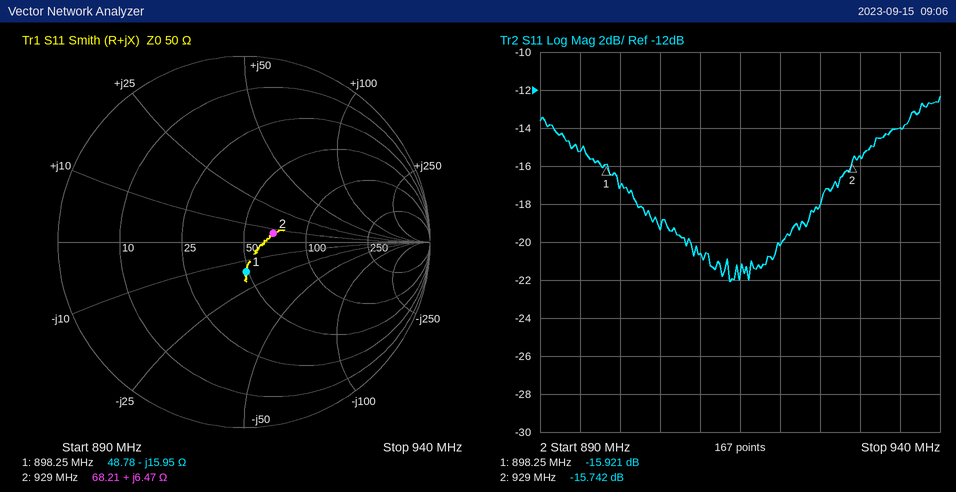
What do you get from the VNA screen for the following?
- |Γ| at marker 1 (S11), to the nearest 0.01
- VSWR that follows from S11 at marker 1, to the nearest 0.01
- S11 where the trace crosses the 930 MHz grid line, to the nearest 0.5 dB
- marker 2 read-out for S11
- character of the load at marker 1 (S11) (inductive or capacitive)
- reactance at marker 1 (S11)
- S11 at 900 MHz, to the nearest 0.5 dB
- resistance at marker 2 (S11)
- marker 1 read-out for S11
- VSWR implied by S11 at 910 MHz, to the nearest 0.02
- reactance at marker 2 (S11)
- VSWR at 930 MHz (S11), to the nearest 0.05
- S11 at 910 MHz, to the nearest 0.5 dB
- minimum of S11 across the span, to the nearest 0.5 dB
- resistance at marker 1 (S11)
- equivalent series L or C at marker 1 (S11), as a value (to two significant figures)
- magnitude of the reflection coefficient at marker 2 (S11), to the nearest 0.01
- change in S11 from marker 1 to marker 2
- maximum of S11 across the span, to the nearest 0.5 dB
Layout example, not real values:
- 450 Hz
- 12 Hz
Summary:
- 0.16
- 1.38
- -15.5 dB
- -15.742 dB
- capacitive
- -15.95 Ω
- -17.0 dB
- 68.21 Ω
- -15.921 dB
- 1.20
- +6.47 Ω
- 1.40
- -20.5 dB
- -22.0 dB
- 48.78 Ω
- 11 pF
- 0.16
- 0.179 dB
- -12.5 dB
